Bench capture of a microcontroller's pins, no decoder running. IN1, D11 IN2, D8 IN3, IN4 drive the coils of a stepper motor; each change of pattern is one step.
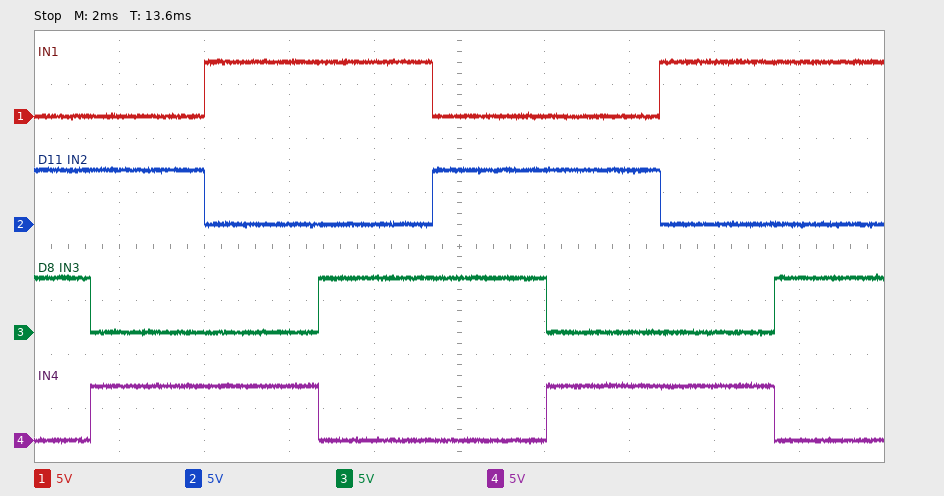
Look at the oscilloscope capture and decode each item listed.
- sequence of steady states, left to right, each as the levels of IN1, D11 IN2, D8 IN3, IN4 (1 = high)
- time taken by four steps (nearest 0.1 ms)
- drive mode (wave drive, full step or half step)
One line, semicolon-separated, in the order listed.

0110 0101 1001 1010 0110 0101 1001 1010; 10.7 ms; full step
